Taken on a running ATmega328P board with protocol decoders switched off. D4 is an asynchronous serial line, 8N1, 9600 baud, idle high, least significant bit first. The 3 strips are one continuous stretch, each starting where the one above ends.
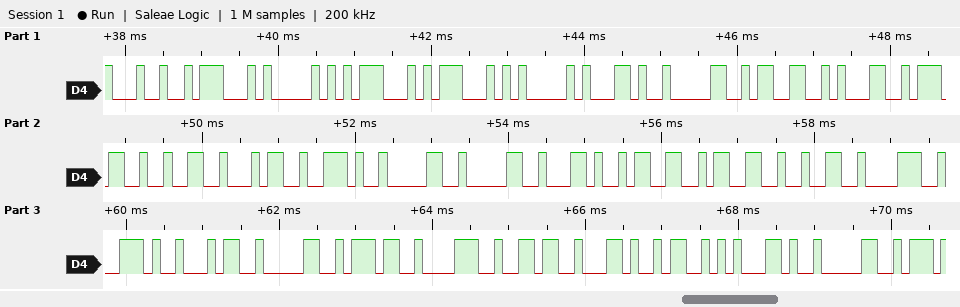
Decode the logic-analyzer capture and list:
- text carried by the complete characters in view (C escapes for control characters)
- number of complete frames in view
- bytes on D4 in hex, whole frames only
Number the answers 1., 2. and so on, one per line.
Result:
1. "$GPGGA,031724.00,3328.40786,S,0"
2. 31
3. 0x24 0x47 0x50 0x47 0x47 0x41 0x2C 0x30 0x33 0x31 0x37 0x32 0x34 0x2E 0x30 0x30 0x2C 0x33 0x33 0x32 0x38 0x2E 0x34 0x30 0x37 0x38 0x36 0x2C 0x53 0x2C 0x30
